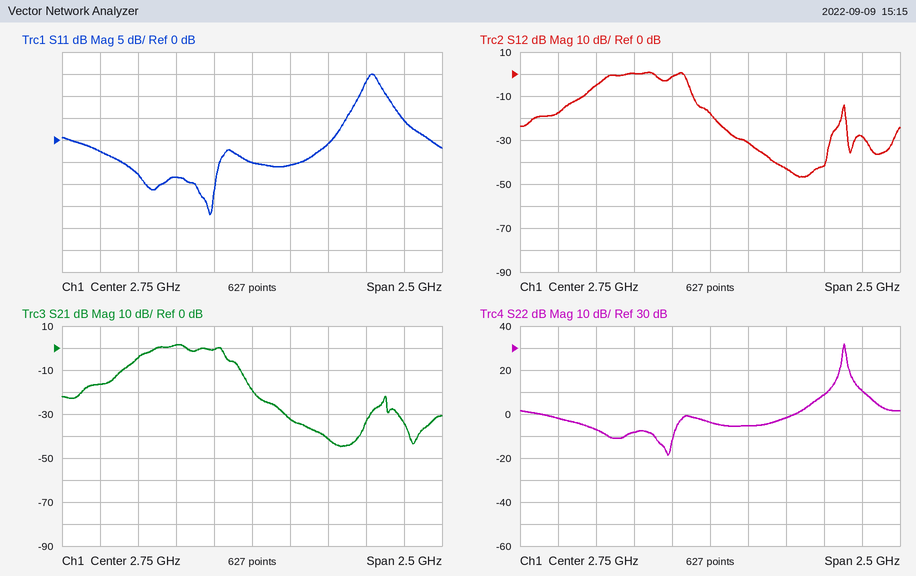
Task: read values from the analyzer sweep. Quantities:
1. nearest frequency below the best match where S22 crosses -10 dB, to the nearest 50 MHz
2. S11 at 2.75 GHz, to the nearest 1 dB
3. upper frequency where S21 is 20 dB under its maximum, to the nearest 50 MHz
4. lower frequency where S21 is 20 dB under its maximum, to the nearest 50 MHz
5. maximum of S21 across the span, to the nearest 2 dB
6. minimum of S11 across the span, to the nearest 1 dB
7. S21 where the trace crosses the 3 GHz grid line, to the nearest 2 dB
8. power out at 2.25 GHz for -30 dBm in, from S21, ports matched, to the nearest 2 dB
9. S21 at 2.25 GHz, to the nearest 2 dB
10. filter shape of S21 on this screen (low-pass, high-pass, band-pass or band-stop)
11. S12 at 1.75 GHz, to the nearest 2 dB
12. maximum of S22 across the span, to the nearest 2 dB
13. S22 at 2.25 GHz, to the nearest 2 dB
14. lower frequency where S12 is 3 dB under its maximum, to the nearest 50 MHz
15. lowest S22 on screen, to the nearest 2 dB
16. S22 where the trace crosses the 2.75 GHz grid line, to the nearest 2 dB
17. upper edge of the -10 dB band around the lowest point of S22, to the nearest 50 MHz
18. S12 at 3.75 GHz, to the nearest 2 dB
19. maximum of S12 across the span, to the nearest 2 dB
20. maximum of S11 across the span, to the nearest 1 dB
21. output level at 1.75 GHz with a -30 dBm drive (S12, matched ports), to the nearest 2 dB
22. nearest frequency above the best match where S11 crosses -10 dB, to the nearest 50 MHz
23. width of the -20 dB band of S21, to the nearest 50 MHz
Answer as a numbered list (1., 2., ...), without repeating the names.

1. 2.40 GHz
2. -5 dB
3. 2.75 GHz
4. 1.65 GHz
5. 2 dB
6. -17 dB
7. -32 dB
8. -28 dBm
9. 2 dB
10. band-pass
11. -18 dB
12. 32 dB
13. -8 dB
14. 2.05 GHz
15. -18 dB
16. -4 dB
17. 2.50 GHz
18. -28 dB
19. 0 dB
20. 15 dB
21. -48 dBm
22. 2.50 GHz
23. 1.10 GHz
